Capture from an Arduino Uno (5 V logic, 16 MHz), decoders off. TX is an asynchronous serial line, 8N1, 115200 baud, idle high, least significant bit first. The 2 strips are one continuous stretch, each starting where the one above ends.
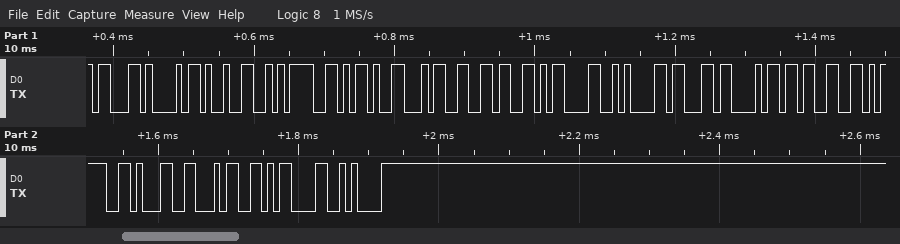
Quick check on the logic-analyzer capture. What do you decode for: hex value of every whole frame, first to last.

0x63 0x68 0x32 0x3D 0x2D 0x34 0x36 0x0D 0x0A 0x63 0x68 0x33 0x3D 0x31 0x34 0x0D 0x0A
